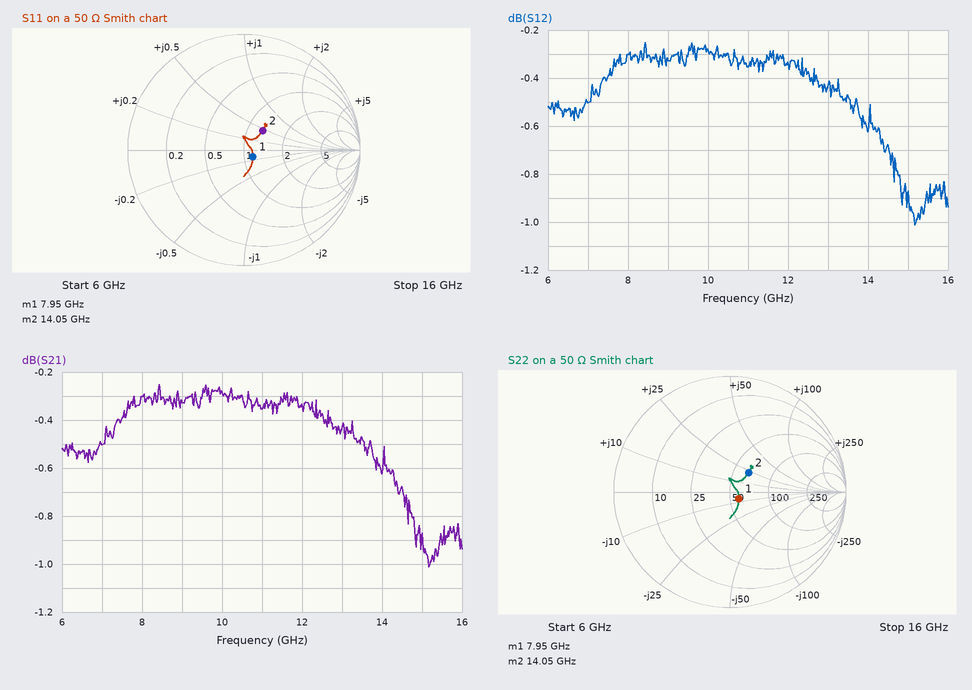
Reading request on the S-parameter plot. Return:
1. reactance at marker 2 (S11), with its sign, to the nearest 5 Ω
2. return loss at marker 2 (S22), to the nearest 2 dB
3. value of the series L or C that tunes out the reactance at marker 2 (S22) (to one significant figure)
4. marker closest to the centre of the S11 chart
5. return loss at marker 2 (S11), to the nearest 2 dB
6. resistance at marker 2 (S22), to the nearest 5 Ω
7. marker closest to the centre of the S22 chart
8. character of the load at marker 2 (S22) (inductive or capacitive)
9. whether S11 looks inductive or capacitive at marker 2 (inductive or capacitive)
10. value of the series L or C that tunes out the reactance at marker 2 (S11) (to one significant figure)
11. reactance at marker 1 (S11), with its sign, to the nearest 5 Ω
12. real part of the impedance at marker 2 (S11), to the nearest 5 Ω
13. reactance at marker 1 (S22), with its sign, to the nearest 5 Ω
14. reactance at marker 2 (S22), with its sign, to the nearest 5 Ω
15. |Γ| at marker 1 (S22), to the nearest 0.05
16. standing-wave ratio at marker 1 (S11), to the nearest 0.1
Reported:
+25 Ω
12 dB
500 fF
marker 1
12 dB
65 Ω
marker 1
inductive
inductive
500 fF
-5 Ω
65 Ω
-5 Ω
+25 Ω
0.10
1.2
